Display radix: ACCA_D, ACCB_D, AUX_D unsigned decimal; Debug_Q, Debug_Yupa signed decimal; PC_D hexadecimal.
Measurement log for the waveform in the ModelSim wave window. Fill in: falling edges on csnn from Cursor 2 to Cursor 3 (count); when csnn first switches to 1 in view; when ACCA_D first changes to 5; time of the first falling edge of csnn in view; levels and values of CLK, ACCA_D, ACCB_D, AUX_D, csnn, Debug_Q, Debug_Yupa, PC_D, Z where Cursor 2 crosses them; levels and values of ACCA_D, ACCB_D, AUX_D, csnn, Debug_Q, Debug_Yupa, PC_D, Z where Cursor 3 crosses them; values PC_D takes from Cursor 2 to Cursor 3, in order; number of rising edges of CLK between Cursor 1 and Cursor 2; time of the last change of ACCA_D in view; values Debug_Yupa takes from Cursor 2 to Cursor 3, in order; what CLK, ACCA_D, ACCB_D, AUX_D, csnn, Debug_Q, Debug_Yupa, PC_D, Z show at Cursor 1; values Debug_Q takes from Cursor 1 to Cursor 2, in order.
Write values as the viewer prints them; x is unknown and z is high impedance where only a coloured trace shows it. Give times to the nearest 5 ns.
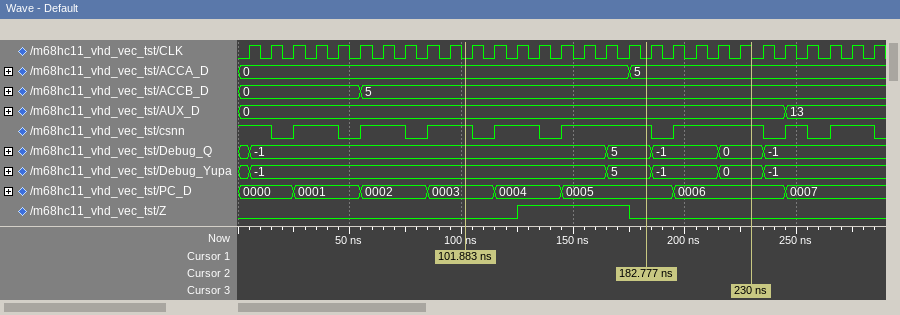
1
25 ns
175 ns
15 ns
CLK=0, ACCA_D=5, ACCB_D=5, AUX_D=0, csnn=1, Debug_Q=5, Debug_Yupa=5, PC_D=0005, Z=0
ACCA_D=5, ACCB_D=5, AUX_D=0, csnn=1, Debug_Q=0, Debug_Yupa=0, PC_D=0006, Z=0
0005, 0006
8
175 ns
5, -1, 0
CLK=0, ACCA_D=0, ACCB_D=5, AUX_D=0, csnn=1, Debug_Q=-1, Debug_Yupa=-1, PC_D=0003, Z=0
-1, 5
